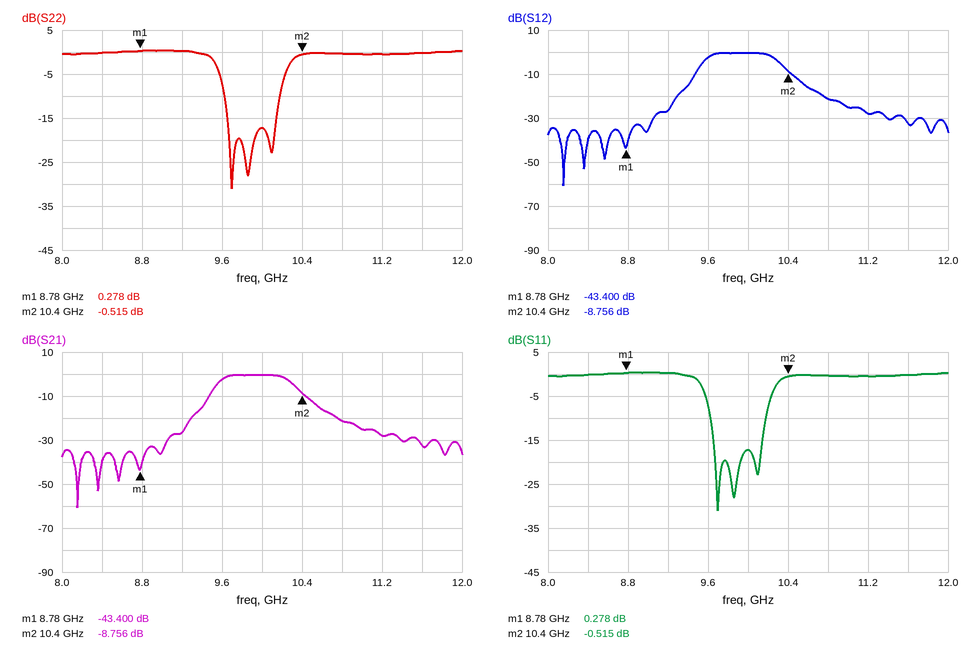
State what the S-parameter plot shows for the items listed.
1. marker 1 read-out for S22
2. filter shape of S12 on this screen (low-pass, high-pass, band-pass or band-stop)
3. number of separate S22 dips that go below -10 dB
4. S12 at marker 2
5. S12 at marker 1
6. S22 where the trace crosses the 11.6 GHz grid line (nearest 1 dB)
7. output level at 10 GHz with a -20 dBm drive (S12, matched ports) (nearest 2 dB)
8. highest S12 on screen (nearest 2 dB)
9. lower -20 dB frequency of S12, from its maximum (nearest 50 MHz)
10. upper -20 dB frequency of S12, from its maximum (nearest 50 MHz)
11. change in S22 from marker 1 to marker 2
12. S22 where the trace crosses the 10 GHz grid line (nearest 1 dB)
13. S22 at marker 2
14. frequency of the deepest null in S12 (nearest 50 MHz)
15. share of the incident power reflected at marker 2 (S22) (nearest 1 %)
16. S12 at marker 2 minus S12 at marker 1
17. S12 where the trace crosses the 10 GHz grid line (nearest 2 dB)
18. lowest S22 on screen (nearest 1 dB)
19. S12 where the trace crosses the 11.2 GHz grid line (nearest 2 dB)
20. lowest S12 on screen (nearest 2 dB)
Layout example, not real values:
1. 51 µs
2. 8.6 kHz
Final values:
1. 0.278 dB
2. band-pass
3. 3
4. -8.756 dB
5. -43.400 dB
6. 0 dB
7. -20 dBm
8. 0 dB
9. 9.30 GHz
10. 10.75 GHz
11. -0.793 dB
12. -17 dB
13. -0.515 dB
14. 8.15 GHz
15. 89 %
16. 34.644 dB
17. 0 dB
18. -31 dB
19. -28 dB
20. -60 dB
